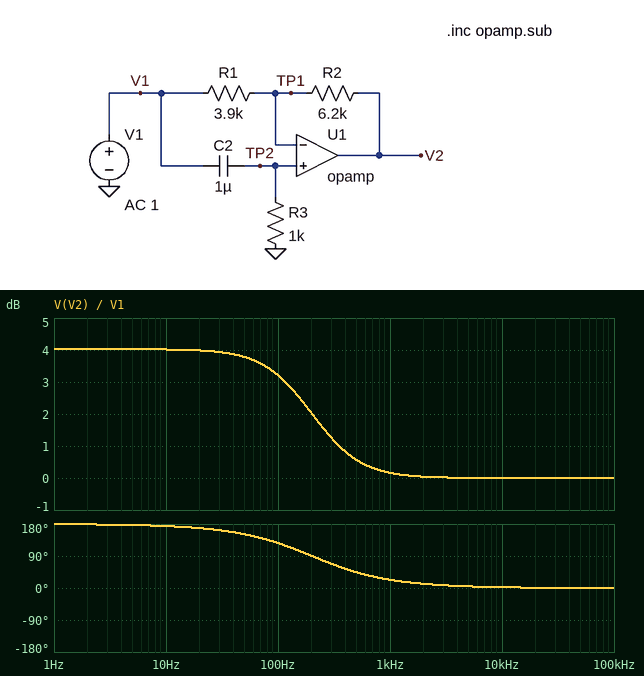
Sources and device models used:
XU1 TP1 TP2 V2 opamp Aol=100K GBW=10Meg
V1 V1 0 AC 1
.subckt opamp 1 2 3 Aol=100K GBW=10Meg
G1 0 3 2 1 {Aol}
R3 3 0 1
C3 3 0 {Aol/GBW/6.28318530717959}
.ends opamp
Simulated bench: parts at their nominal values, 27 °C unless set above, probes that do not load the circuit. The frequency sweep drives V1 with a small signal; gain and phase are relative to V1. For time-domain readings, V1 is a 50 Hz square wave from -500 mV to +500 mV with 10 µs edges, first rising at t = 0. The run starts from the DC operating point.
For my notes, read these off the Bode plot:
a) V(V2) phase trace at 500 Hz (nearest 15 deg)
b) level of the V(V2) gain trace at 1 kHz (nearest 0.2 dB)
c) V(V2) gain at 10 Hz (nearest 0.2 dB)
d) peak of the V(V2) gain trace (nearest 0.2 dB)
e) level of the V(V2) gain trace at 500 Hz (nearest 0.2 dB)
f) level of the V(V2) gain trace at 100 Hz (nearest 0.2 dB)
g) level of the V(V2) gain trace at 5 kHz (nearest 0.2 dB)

45 deg
0.2 dB
4.0 dB
4.0 dB
0.6 dB
3.2 dB
0 dB
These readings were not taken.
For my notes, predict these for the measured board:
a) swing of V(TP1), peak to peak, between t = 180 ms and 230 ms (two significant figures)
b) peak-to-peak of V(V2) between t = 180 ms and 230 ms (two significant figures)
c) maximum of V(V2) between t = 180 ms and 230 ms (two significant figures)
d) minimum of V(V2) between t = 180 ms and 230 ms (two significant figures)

2.0 V
3.6 V
1.8 V
-1.8 V
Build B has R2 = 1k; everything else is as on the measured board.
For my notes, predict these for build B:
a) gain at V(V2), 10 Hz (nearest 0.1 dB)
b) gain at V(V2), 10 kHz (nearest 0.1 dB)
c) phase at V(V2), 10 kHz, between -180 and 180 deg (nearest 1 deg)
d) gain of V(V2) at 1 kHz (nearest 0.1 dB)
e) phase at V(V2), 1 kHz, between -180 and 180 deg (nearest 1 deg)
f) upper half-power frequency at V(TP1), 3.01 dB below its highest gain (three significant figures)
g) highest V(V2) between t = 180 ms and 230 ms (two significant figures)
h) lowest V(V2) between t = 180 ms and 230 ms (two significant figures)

-11.6 dB
0 dB
1 deg
-0.1 dB
11 deg
8.31 MHz
1.1 V
-1.1 V
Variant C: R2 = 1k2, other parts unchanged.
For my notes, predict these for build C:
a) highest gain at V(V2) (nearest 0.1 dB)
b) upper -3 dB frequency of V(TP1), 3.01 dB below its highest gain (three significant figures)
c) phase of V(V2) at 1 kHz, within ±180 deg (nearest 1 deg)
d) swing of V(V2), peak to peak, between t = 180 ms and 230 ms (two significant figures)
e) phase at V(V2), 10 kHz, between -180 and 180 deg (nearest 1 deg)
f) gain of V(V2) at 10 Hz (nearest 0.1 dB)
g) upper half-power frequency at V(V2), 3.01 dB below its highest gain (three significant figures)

0 dB
8.11 MHz
12 deg
2.3 V
1 deg
-10.1 dB
7.65 MHz
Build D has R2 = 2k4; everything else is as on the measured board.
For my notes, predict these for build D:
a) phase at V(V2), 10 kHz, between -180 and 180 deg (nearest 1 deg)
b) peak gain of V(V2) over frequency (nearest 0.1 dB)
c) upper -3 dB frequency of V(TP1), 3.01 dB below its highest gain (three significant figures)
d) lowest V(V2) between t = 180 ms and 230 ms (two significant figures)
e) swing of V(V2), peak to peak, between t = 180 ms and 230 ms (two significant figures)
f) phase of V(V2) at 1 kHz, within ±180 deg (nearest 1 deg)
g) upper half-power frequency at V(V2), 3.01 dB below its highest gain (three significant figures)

1 deg
0 dB
7.35 MHz
-1.3 V
2.6 V
15 deg
6.19 MHz
